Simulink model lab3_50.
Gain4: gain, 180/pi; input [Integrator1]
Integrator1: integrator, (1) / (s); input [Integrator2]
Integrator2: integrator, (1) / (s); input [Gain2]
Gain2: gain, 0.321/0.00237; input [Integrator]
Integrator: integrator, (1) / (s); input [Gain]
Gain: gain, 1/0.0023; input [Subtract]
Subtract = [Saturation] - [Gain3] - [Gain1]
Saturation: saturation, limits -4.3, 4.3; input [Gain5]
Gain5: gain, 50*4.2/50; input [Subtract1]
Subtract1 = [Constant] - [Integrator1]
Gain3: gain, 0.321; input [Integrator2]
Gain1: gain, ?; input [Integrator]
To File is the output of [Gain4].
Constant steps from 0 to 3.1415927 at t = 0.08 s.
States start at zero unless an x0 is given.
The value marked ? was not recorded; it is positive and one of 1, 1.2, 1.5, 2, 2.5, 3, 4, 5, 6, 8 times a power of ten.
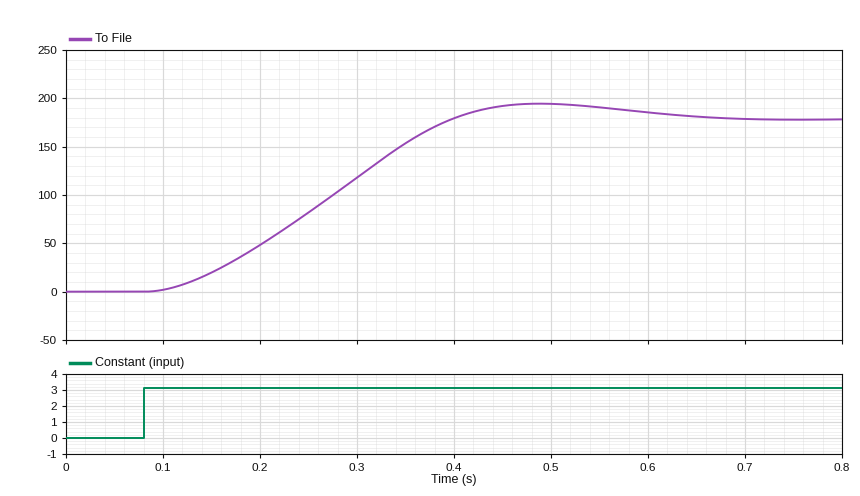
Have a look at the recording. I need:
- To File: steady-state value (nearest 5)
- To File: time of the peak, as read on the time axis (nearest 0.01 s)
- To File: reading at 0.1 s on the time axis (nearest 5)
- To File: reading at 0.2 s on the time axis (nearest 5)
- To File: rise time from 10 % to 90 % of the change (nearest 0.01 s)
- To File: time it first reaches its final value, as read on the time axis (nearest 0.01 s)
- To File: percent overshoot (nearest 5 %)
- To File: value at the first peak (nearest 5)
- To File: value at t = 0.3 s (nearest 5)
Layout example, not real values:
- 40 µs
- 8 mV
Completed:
- 180
- 0.49 s
- 0
- 50
- 0.22 s
- 0.40 s
- 10 %
- 195
- 120
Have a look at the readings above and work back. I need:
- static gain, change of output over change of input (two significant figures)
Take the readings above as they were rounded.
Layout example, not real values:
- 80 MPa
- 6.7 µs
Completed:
- 57
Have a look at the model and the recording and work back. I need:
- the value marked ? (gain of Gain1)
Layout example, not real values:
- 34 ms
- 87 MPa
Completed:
- 3
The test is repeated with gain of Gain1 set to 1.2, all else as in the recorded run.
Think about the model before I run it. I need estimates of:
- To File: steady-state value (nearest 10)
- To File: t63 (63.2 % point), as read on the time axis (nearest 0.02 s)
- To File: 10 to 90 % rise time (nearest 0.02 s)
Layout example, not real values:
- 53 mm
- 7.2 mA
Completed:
- 180
- 0.26 s
- 0.20 s
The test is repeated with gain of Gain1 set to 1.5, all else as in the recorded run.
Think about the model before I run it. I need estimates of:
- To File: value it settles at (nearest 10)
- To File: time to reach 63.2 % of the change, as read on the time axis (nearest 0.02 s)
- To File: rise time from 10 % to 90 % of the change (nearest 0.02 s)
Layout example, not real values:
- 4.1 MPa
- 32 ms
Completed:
- 180
- 0.26 s
- 0.20 s
